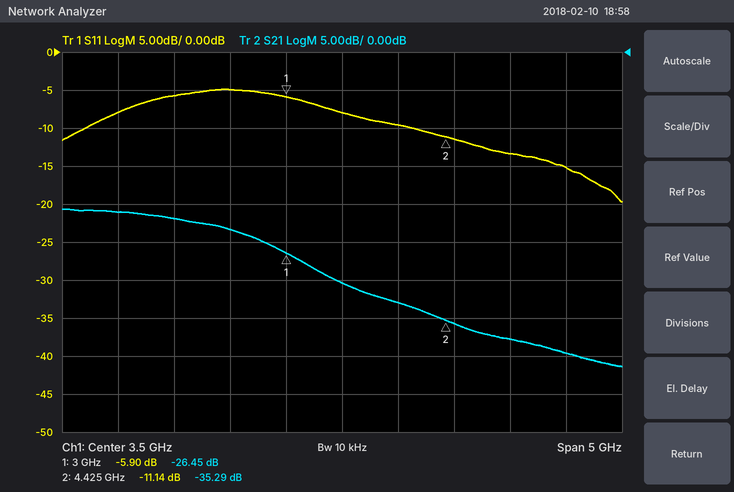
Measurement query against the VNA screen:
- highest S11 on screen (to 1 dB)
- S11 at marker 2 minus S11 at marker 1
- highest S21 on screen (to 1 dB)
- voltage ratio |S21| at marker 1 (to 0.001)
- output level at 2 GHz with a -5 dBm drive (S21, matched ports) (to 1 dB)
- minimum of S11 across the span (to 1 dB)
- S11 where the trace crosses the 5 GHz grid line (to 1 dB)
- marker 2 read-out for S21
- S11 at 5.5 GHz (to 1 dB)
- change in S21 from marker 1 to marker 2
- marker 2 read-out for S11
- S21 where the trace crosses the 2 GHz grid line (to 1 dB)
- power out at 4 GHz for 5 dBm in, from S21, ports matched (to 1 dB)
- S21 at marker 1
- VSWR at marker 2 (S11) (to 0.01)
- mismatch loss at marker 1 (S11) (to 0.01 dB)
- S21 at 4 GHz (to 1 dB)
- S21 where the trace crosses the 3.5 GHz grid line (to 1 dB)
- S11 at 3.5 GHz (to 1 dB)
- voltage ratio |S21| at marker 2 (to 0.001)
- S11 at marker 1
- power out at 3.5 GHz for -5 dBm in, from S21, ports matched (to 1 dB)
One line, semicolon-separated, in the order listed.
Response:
-5 dB; -5.24 dB; -21 dB; 0.048; -27 dBm; -20 dB; -13 dB; -35.29 dB; -15 dB; -8.84 dB; -11.14 dB; -22 dB; -28 dBm; -26.45 dB; 1.77; 1.29 dB; -33 dB; -30 dB; -8 dB; 0.017; -5.90 dB; -35 dBm
